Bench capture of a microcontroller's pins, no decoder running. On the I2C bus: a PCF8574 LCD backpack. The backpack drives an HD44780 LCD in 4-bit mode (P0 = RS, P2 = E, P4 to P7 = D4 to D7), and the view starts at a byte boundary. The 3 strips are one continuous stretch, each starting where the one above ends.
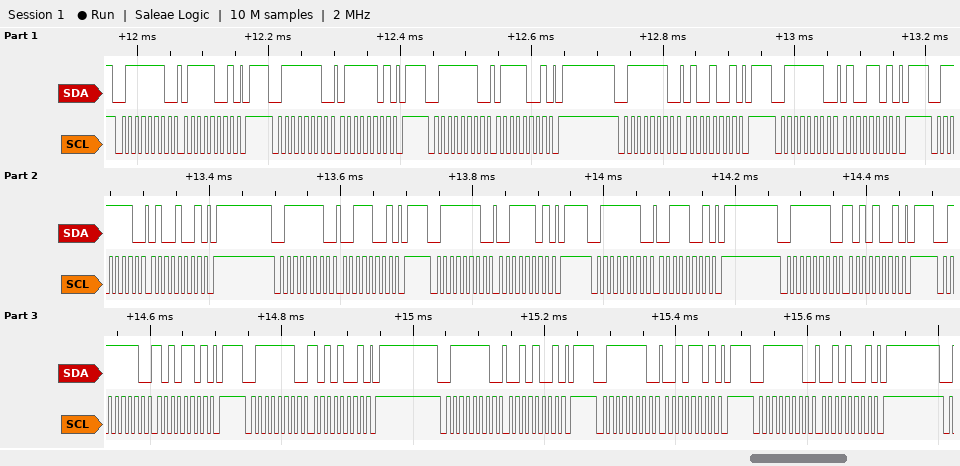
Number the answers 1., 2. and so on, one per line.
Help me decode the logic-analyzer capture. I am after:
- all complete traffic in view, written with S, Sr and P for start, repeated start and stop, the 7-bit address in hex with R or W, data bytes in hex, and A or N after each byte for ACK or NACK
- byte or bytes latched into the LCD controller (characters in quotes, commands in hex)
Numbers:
1. S 3FW A 79 A P S 3FW A 7D A P S 3FW A 79 A P S 3FW A 49 A P S 3FW A 4D A P S 3FW A 49 A P S 3FW A 39 A P S 3FW A 3D A P S 3FW A 39 A P S 3FW A A9 A P S 3FW A AD A P S 3FW A A9 A P S 3FW A 29 A P S 3FW A 2D A P S 3FW A 29 A P
2. 't' ':'
